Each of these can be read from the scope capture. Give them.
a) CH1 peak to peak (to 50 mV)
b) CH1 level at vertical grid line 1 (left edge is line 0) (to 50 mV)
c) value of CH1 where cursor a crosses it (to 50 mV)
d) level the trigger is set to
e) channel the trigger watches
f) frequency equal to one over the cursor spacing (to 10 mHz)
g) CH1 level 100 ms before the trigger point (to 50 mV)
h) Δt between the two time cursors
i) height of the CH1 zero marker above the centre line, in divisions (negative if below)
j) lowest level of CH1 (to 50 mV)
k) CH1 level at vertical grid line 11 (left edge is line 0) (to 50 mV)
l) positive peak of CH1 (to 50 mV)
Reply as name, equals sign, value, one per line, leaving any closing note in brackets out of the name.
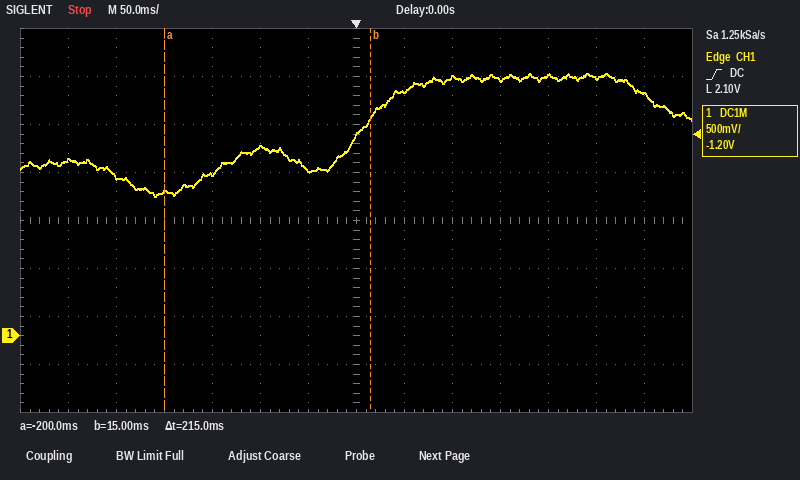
CH1 peak to peak = 1.30 V
CH1 level at vertical grid line 1 (left edge is line 0) = 1.85 V
value of CH1 where cursor a crosses it = 1.50 V
level the trigger is set to = 2.10 V
channel the trigger watches = CH1
frequency equal to one over the cursor spacing = 4.65 Hz
CH1 level 100 ms before the trigger point = 1.95 V
Δt between the two time cursors = 215 ms
height of the CH1 zero marker above the centre line, in divisions = -2.4 div
lowest level of CH1 = 1.45 V
CH1 level at vertical grid line 11 (left edge is line 0) = 2.70 V
positive peak of CH1 = 2.75 V
